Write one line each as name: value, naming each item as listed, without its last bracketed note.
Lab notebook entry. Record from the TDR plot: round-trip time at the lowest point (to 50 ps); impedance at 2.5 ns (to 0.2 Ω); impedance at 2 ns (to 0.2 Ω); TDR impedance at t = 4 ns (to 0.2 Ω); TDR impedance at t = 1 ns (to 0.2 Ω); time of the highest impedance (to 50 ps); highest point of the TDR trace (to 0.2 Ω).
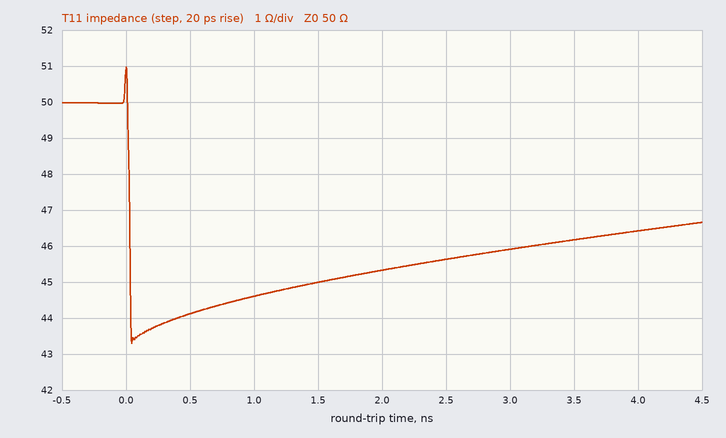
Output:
round-trip time at the lowest point: 50 ps
impedance at 2.5 ns: 45.6 Ω
impedance at 2 ns: 45.4 Ω
TDR impedance at t = 4 ns: 46.4 Ω
TDR impedance at t = 1 ns: 44.6 Ω
time of the highest impedance: 0 ps
highest point of the TDR trace: 51.0 Ω
